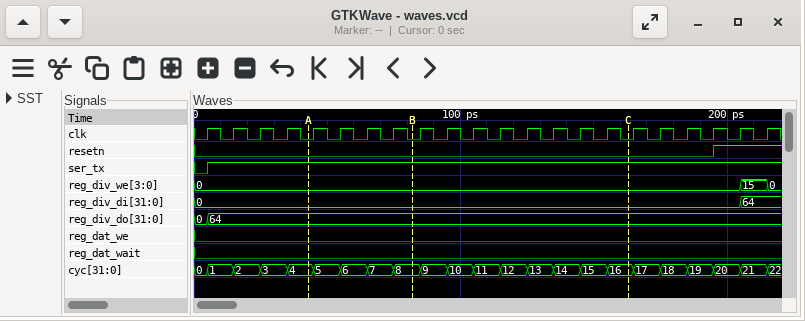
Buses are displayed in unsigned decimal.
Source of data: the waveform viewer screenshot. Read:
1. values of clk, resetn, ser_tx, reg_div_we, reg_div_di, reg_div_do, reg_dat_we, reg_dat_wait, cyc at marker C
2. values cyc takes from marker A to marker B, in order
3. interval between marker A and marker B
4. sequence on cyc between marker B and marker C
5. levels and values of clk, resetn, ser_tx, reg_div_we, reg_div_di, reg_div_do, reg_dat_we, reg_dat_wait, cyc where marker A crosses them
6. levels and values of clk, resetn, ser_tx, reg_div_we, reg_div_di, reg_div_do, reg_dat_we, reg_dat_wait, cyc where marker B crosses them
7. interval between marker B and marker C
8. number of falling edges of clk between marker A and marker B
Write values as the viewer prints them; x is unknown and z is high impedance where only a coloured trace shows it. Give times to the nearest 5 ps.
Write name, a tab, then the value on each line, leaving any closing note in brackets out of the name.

values of clk, resetn, ser_tx, reg_div_we, reg_div_di, reg_div_do, reg_dat_we, reg_dat_wait, cyc at marker C	clk=0, resetn=0, ser_tx=1, reg_div_we=0, reg_div_di=0, reg_div_do=64, reg_dat_we=0, reg_dat_wait=0, cyc=16
values cyc takes from marker A to marker B, in order	4, 5, 6, 7, 8
interval between marker A and marker B	40 ps
sequence on cyc between marker B and marker C	8, 9, 10, 11, 12, 13, 14, 15, 16
levels and values of clk, resetn, ser_tx, reg_div_we, reg_div_di, reg_div_do, reg_dat_we, reg_dat_wait, cyc where marker A crosses them	clk=0, resetn=0, ser_tx=1, reg_div_we=0, reg_div_di=0, reg_div_do=64, reg_dat_we=0, reg_dat_wait=0, cyc=4
levels and values of clk, resetn, ser_tx, reg_div_we, reg_div_di, reg_div_do, reg_dat_we, reg_dat_wait, cyc where marker B crosses them	clk=0, resetn=0, ser_tx=1, reg_div_we=0, reg_div_di=0, reg_div_do=64, reg_dat_we=0, reg_dat_wait=0, cyc=8
interval between marker B and marker C	80 ps
number of falling edges of clk between marker A and marker B	4
